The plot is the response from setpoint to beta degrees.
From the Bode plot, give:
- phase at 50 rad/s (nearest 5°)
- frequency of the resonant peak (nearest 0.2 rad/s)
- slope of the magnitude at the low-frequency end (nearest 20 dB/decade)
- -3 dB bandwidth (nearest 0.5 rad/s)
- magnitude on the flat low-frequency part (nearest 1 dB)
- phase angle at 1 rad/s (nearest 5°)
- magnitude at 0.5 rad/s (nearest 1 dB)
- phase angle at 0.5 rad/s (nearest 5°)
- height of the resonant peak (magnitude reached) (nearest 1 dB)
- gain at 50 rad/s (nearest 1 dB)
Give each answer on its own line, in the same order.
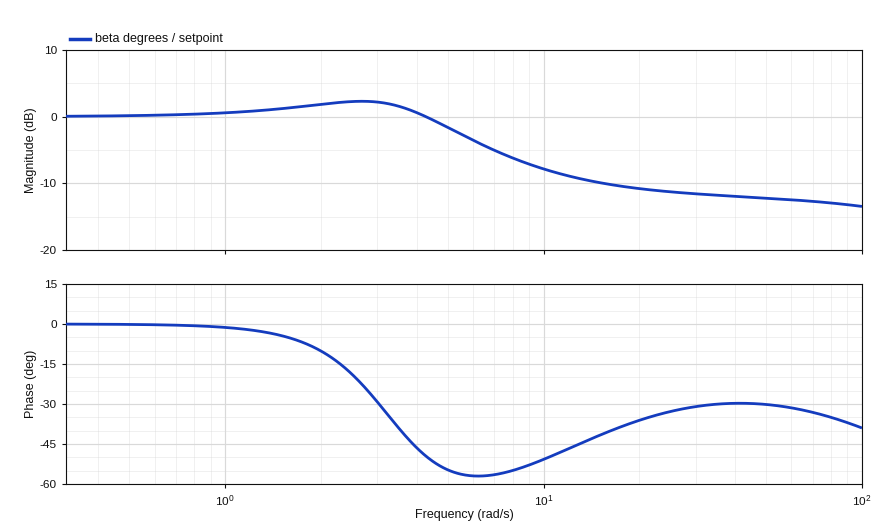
-30°
2.6 rad/s
0 dB/decade
5.5 rad/s
0 dB
0°
0 dB
0°
2 dB
-12 dB
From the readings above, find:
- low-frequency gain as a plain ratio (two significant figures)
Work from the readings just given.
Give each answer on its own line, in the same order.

1.0
